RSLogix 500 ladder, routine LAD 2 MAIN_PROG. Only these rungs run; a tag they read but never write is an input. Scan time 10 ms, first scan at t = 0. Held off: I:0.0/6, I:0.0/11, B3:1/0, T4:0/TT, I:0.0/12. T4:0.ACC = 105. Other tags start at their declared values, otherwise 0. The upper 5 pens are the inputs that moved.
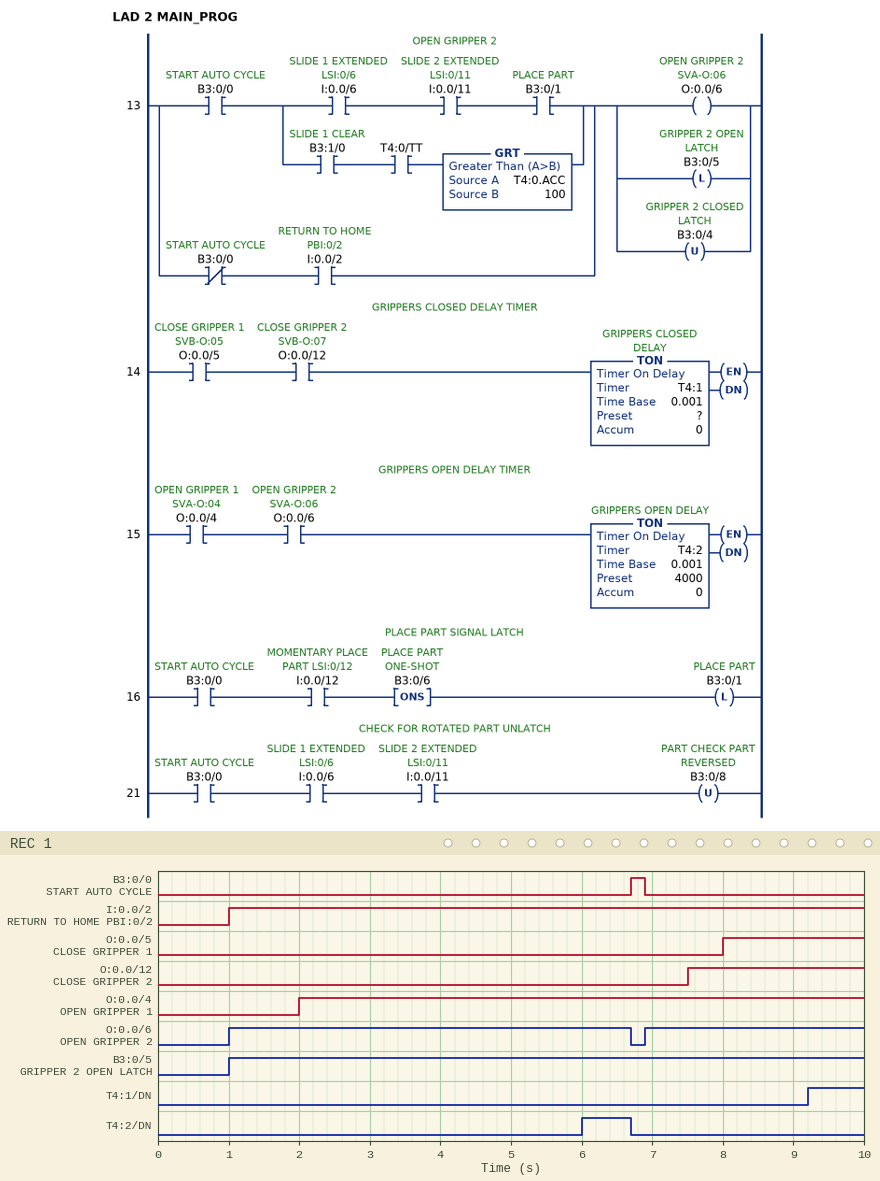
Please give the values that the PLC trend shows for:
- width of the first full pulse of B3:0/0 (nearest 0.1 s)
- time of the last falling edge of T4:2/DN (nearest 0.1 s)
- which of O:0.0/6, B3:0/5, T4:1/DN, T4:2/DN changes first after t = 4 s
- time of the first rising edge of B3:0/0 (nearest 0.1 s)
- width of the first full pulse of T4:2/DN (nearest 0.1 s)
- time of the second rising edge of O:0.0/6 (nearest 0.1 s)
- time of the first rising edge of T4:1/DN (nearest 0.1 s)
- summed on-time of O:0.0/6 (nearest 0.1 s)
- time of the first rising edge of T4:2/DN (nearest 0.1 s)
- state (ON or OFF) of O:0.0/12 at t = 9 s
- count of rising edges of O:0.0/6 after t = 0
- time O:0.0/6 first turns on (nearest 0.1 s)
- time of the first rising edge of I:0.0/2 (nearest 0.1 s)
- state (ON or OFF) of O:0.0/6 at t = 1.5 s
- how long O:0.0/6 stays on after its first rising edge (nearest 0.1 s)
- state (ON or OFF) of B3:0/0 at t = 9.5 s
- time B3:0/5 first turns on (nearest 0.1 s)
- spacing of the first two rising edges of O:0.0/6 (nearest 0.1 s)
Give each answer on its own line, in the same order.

0.2 s
6.7 s
T4:2/DN
6.7 s
0.7 s
6.9 s
9.2 s
8.8 s
6.0 s
ON
2
1.0 s
1.0 s
ON
5.7 s
OFF
1.0 s
5.9 s
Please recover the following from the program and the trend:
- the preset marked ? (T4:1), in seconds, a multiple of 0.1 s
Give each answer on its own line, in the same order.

1.2 s
